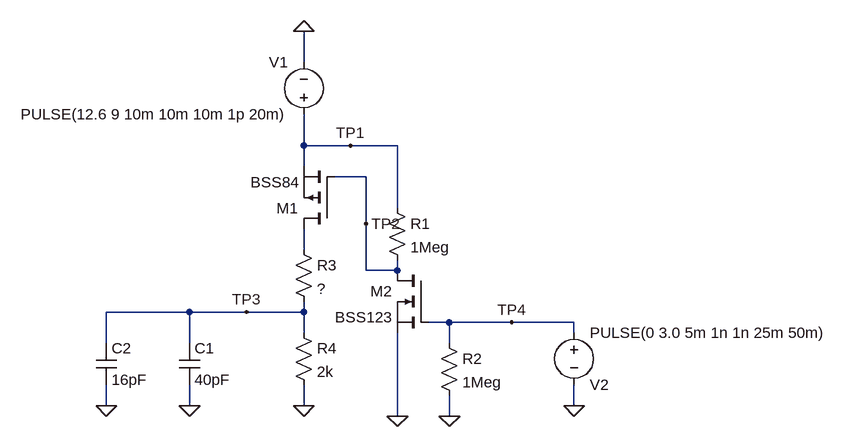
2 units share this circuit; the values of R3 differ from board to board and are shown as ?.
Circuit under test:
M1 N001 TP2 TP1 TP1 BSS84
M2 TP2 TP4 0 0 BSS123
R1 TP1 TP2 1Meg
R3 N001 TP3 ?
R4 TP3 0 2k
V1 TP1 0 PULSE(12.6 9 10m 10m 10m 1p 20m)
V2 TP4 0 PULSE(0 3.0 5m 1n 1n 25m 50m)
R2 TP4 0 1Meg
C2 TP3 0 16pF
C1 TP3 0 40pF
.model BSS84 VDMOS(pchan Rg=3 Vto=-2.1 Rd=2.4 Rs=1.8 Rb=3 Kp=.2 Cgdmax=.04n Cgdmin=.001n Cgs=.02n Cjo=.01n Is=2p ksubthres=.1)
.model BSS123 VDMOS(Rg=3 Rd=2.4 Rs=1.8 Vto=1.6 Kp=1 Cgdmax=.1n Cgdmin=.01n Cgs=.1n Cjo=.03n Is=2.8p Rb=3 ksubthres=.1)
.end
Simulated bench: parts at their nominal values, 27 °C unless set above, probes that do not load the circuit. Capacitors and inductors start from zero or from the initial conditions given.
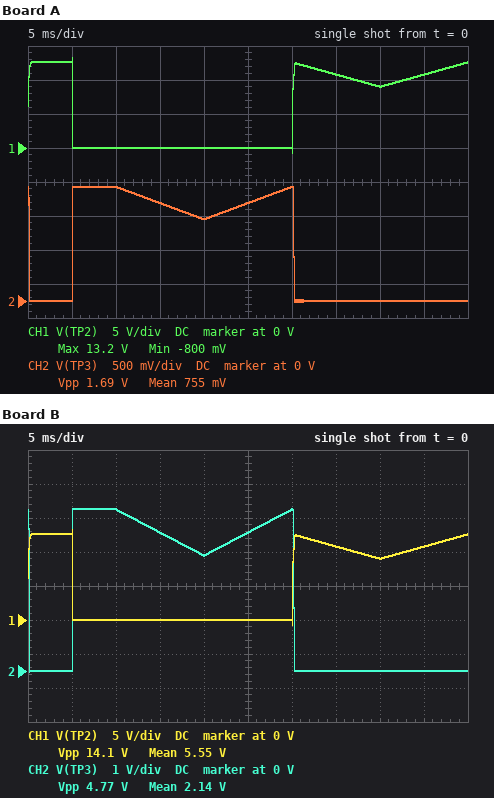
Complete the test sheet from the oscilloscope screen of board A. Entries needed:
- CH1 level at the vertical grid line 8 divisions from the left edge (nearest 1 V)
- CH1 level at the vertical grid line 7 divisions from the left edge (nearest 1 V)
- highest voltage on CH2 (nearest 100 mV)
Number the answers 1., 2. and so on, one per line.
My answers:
1. 9 V
2. 11 V
3. 1.7 V
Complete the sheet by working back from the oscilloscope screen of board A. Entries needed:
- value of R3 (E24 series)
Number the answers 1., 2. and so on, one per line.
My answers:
1. 13 kΩ
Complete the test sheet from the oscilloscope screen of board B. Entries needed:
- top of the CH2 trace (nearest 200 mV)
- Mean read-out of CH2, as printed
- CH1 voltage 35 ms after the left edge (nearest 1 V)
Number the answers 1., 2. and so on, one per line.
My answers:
1. 4.8 V
2. 2.14 V
3. 11 V
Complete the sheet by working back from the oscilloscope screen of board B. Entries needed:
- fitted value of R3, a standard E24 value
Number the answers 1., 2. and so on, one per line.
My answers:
1. 3.3 kΩ
